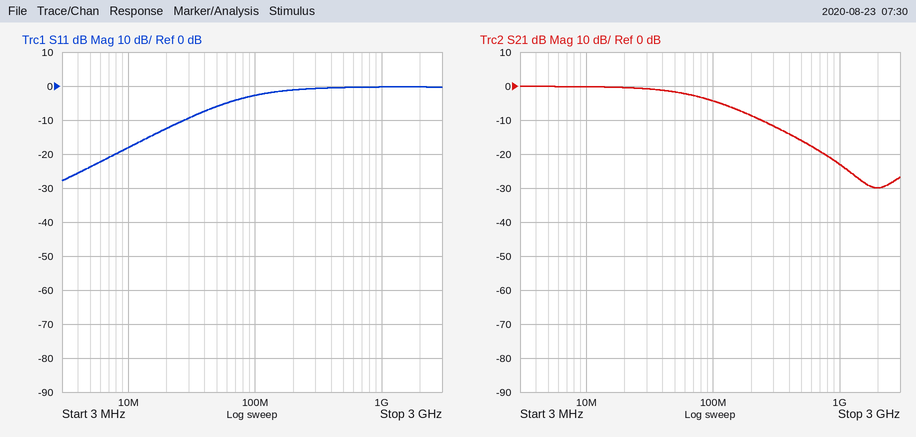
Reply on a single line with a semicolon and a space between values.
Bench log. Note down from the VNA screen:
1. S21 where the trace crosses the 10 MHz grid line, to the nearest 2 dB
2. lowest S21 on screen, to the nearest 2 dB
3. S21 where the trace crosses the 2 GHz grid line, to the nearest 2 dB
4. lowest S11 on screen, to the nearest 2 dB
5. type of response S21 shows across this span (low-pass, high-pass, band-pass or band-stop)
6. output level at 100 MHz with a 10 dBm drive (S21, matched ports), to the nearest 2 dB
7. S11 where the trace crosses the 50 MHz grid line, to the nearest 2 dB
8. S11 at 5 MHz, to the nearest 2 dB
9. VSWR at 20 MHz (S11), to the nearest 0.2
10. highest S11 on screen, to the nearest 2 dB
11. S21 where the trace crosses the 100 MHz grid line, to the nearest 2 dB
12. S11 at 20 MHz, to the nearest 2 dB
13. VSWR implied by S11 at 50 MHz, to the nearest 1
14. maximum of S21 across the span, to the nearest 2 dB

0 dB; -30 dB; -30 dB; -28 dB; low-pass; 6 dBm; -6 dB; -24 dB; 1.6; 0 dB; -4 dB; -12 dB; 3; 0 dB
